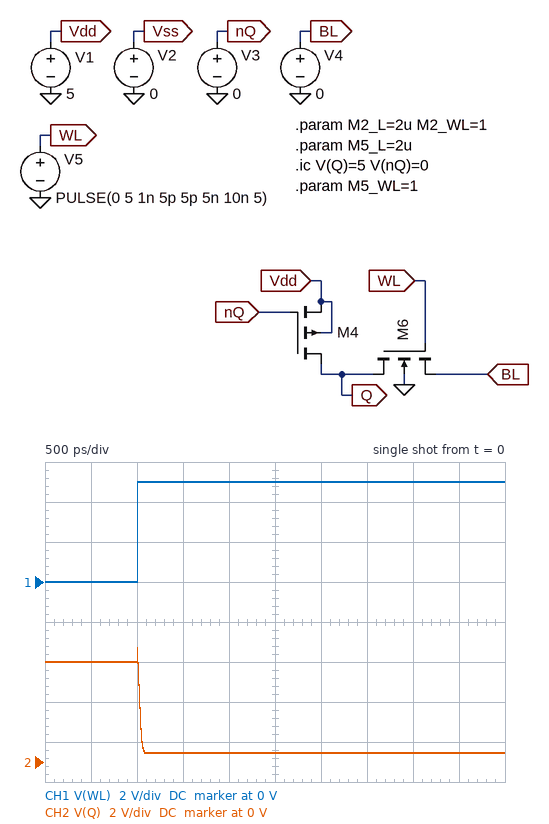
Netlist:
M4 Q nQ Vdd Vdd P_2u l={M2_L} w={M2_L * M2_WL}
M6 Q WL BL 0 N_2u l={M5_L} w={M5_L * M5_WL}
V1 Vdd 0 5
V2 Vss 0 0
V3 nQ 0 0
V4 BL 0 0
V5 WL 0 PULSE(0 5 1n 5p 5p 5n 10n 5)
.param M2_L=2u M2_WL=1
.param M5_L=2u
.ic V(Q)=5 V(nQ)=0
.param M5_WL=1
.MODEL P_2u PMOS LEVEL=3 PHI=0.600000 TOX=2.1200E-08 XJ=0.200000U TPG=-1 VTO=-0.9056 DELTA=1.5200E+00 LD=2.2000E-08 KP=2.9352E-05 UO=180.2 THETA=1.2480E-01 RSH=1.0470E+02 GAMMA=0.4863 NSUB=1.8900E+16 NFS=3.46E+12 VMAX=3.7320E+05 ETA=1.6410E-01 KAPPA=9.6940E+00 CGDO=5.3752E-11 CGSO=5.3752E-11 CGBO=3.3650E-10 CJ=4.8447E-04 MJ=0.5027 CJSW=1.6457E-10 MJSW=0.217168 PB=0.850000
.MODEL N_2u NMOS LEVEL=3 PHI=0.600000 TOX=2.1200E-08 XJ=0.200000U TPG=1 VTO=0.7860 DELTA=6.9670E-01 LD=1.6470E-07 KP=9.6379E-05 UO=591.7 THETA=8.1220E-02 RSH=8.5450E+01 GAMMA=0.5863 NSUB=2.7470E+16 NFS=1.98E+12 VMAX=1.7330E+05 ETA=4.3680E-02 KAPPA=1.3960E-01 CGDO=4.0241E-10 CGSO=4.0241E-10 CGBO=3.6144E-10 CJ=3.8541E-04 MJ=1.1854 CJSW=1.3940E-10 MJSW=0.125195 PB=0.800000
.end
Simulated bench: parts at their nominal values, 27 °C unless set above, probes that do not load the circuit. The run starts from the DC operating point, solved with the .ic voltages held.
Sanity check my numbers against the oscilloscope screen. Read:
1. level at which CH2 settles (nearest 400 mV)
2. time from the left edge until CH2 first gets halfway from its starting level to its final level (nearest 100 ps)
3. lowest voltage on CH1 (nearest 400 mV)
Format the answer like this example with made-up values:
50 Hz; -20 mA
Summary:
400 mV; 1.0 ns; 0 V
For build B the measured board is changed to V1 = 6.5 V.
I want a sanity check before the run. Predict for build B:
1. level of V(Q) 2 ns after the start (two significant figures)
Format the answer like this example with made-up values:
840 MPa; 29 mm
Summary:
770 mV
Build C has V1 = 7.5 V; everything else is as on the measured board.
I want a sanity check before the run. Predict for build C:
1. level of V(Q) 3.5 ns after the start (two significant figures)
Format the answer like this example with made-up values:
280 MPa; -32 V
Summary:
1.1 V
